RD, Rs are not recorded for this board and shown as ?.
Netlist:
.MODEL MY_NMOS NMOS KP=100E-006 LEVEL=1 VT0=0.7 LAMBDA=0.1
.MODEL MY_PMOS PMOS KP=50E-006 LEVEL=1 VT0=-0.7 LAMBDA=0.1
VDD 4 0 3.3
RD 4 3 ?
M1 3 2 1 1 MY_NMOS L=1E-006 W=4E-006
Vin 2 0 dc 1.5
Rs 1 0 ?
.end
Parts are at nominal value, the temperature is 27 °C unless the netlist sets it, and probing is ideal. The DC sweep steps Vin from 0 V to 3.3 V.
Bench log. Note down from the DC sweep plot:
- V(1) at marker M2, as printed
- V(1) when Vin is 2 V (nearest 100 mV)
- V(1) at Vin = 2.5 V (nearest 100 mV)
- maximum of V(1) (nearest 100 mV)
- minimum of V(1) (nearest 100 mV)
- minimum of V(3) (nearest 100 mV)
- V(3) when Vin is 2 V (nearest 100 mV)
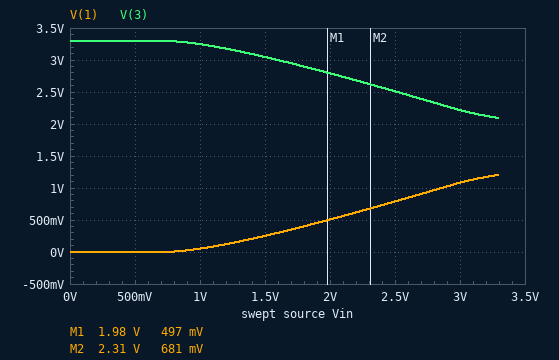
681 mV
500 mV
800 mV
1.2 V
0 V
2.1 V
2.8 V
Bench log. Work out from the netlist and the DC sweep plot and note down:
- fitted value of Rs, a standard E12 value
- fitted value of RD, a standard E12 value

3.3 kΩ
3.3 kΩ
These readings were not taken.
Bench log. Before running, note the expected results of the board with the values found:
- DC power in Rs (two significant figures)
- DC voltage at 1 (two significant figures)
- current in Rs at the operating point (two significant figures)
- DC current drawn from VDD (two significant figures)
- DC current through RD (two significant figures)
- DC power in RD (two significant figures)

19 µW
250 mV
77 µA
77 µA
77 µA
19 µW
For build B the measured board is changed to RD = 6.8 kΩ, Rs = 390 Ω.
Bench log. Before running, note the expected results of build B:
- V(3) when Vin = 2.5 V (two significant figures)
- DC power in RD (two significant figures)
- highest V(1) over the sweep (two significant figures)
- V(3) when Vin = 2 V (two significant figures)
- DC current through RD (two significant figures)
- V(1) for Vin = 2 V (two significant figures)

790 mV
130 µW
160 mV
1.2 V
140 µA
120 mV
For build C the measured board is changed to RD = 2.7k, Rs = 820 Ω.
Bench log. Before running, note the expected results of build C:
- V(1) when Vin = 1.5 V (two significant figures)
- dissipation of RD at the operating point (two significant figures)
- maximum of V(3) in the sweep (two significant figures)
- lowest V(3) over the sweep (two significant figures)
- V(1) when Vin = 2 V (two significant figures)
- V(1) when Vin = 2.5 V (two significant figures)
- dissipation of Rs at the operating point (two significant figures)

100 mV
42 µW
3.3 V
1.5 V
230 mV
380 mV
13 µW
